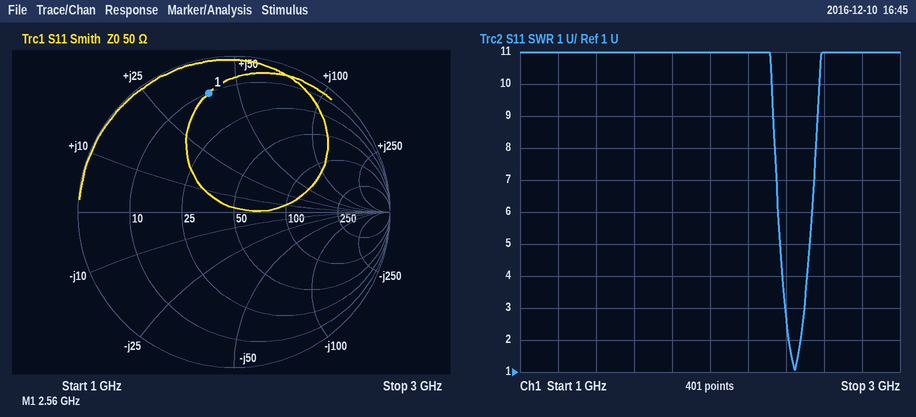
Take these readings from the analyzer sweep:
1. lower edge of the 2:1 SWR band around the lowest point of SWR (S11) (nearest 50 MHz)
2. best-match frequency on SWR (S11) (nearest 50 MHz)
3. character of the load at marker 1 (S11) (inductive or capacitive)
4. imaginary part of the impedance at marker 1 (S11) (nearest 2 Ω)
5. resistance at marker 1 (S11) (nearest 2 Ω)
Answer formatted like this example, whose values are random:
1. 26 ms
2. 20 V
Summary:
1. 2.40 GHz
2. 2.45 GHz
3. inductive
4. +40 Ω
5. 10 Ω
